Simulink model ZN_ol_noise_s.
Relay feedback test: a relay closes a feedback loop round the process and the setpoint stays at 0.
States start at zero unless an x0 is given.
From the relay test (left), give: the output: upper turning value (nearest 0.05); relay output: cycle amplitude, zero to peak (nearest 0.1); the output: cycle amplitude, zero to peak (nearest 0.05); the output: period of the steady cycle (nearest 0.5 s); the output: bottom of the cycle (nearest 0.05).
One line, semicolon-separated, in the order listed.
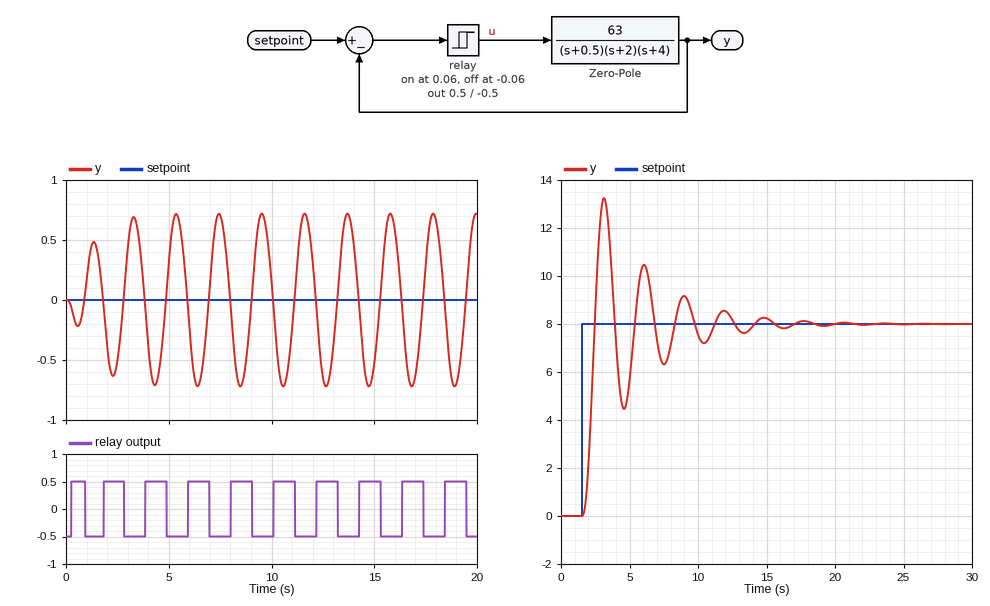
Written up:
0.70; 0.5; 0.70; 2.0 s; -0.70
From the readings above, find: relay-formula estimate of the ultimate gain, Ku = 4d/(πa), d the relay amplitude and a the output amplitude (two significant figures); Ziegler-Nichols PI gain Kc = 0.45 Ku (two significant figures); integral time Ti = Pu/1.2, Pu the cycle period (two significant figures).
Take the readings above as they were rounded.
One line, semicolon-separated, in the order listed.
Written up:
0.91; 0.41; 1.7 s
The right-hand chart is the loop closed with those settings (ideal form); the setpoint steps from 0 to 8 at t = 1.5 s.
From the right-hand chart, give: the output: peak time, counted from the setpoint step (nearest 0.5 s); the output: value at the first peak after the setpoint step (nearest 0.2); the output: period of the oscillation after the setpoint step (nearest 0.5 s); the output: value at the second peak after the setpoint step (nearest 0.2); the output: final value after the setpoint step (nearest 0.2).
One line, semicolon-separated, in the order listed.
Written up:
1.5 s; 13.2; 3.0 s; 10.4; 8.0
